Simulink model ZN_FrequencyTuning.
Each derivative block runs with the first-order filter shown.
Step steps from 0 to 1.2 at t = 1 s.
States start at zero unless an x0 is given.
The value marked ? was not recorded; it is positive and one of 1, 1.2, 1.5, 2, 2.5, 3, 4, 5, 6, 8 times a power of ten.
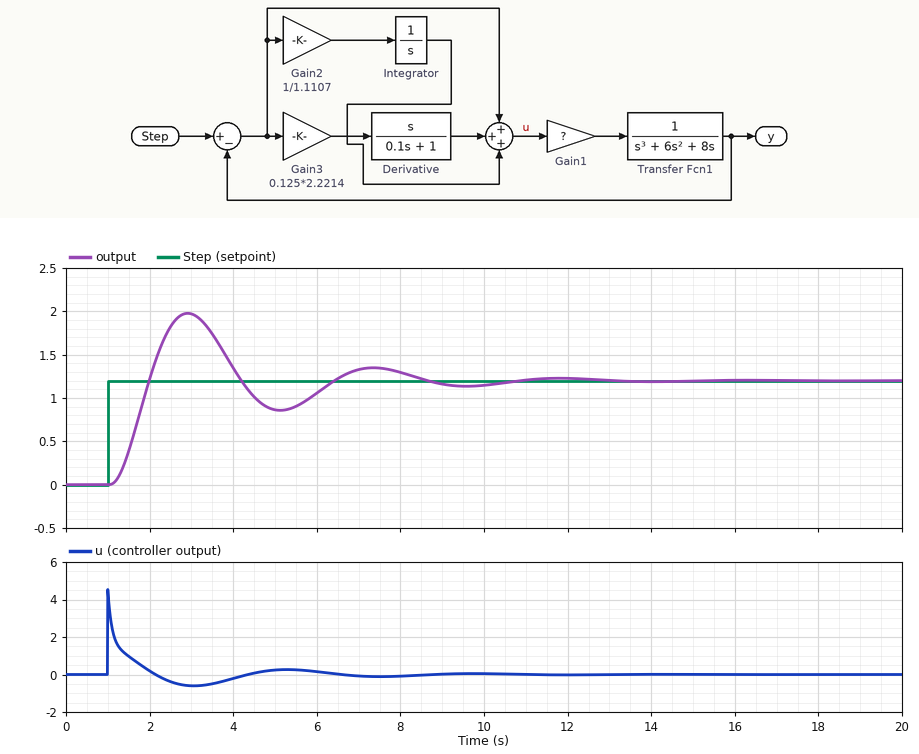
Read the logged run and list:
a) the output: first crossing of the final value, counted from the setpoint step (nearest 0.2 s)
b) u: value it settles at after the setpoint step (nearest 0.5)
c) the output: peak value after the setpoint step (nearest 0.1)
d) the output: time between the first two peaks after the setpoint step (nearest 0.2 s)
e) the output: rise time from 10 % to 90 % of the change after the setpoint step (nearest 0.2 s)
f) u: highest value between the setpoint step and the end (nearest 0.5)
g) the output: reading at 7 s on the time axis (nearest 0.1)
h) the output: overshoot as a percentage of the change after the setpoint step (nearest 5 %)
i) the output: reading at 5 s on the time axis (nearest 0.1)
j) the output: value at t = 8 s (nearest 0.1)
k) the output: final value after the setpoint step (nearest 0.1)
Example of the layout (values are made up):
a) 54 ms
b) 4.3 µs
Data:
a) 1.0 s
b) 0.0
c) 2.0
d) 4.4 s
e) 0.6 s
f) 4.5
g) 1.3
h) 65 %
i) 0.9
j) 1.3
k) 1.2
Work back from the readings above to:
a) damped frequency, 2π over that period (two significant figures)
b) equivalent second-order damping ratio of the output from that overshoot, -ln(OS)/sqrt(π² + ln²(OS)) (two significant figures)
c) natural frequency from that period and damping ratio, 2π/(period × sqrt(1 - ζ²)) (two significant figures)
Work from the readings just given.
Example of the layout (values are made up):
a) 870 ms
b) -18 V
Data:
a) 1.4 rad/s
b) 0.14
c) 1.4 rad/s
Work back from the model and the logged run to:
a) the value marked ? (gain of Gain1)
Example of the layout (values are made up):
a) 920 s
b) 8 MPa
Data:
a) 15
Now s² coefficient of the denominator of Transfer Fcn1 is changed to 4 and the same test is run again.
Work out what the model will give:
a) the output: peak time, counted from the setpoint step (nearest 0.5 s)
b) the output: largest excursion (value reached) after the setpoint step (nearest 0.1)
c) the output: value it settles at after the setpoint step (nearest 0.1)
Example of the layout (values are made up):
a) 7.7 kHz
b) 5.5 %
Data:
a) 1.5 s
b) 1.9
c) 1.2
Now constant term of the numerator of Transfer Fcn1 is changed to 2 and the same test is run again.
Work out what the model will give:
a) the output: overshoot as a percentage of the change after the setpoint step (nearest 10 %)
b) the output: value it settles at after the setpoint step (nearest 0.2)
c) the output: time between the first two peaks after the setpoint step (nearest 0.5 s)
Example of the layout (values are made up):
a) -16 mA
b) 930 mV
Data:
a) 70 %
b) 1.2
c) 2.5 s
